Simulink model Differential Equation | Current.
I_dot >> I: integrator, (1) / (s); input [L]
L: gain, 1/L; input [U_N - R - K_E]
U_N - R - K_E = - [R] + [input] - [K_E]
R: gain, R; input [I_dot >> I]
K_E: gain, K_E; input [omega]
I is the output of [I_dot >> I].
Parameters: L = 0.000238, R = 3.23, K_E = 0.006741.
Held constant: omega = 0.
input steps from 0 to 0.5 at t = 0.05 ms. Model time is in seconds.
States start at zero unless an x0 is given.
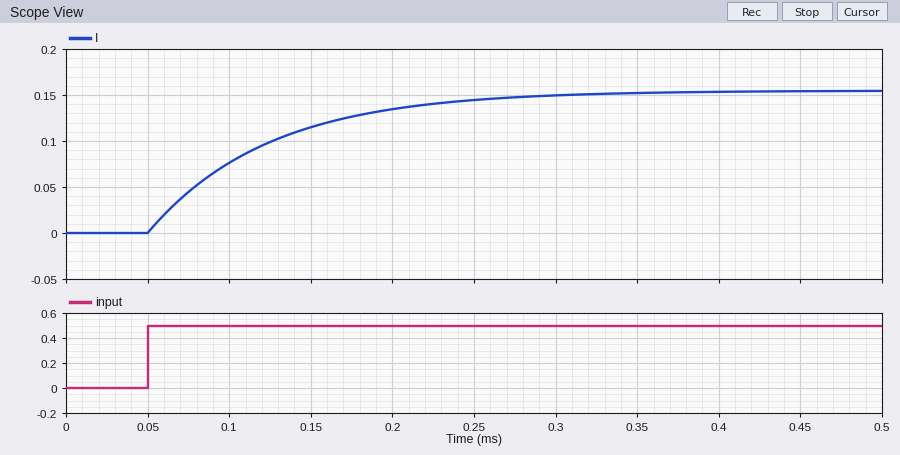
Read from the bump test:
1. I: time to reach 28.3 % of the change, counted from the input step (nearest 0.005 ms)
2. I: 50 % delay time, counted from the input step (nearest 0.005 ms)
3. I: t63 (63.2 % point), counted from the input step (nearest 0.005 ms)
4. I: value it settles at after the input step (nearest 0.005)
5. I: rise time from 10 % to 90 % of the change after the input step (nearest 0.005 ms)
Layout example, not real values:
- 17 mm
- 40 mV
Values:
- 0.025 ms
- 0.050 ms
- 0.075 ms
- 0.155
- 0.160 ms
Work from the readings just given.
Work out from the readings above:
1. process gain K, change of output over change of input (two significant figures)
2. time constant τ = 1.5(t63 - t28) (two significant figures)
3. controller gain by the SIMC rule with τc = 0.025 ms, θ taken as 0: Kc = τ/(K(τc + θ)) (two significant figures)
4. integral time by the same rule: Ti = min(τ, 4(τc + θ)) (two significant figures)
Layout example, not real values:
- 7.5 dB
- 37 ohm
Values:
- 0.31
- 0.075 ms
- 9.7
- 0.075 ms
